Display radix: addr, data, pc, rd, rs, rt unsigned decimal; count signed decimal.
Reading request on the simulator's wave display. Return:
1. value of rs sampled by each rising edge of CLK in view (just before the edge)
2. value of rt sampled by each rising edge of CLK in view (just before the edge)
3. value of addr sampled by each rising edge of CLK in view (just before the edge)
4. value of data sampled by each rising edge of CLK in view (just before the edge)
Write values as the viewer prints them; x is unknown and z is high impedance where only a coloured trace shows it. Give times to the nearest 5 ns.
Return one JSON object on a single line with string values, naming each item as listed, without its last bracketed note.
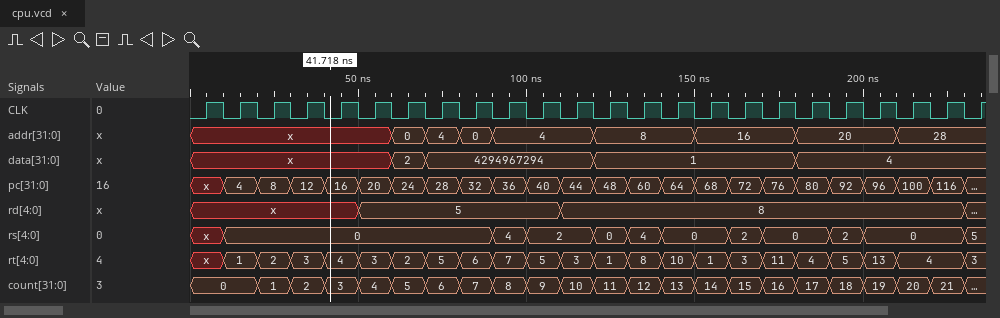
{"value of rs sampled by each rising edge of CLK in view": "x, 0, 0, 0, 0, 0, 0, 0, 0, 4, 2, 2, 0, 4, 0, 0, 2, 0, 0, 2, 0, 0, 0, 5", "value of rt sampled by each rising edge of CLK in view": "x, 1, 2, 3, 4, 3, 2, 5, 6, 7, 5, 3, 1, 8, 10, 1, 3, 11, 4, 5, 13, 4, 4, 3", "value of addr sampled by each rising edge of CLK in view": "x, x, x, x, x, x, 0, 4, 0, 4, 4, 4, 8, 8, 8, 16, 16, 16, 20, 20, 20, 28, 28, 28", "value of data sampled by each rising edge of CLK in view": "x, x, x, x, x, x, 2, 4294967294, 4294967294, 4294967294, 4294967294, 4294967294, 1, 1, 1, 1, 1, 1, 4, 4, 4, 4, 4, 4"}
